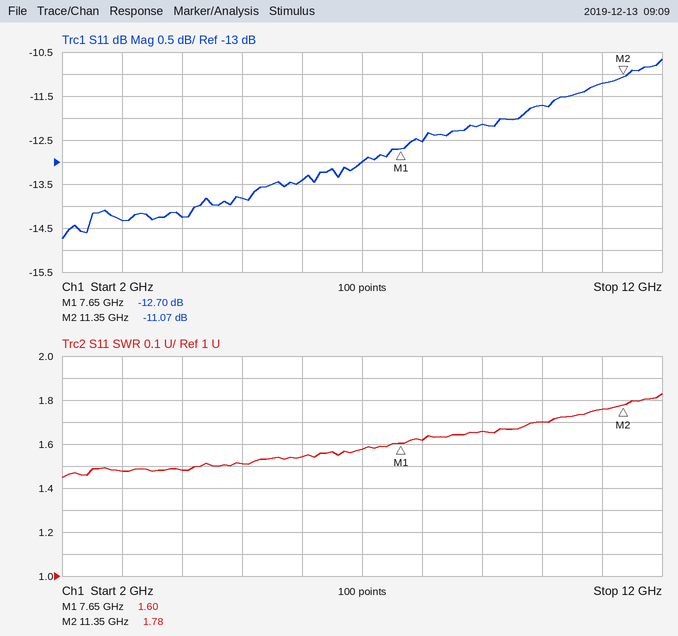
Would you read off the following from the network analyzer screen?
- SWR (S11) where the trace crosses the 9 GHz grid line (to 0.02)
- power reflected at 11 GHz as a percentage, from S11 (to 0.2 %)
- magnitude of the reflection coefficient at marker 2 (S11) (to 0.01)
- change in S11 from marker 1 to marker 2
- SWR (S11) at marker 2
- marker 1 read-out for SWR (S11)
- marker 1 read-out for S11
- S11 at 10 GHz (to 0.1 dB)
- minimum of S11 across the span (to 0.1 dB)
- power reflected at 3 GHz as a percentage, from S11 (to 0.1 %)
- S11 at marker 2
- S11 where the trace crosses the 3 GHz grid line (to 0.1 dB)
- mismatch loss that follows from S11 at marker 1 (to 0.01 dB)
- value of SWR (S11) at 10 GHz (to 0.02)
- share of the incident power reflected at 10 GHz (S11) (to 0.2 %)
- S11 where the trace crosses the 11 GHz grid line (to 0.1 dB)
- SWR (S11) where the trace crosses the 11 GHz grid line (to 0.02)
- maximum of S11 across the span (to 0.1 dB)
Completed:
1.66
7.6 %
0.28
1.63 dB
1.78
1.60
-12.70 dB
-11.7 dB
-14.7 dB
3.7 %
-11.07 dB
-14.3 dB
0.24 dB
1.70
6.8 %
-11.2 dB
1.76
-10.7 dB
